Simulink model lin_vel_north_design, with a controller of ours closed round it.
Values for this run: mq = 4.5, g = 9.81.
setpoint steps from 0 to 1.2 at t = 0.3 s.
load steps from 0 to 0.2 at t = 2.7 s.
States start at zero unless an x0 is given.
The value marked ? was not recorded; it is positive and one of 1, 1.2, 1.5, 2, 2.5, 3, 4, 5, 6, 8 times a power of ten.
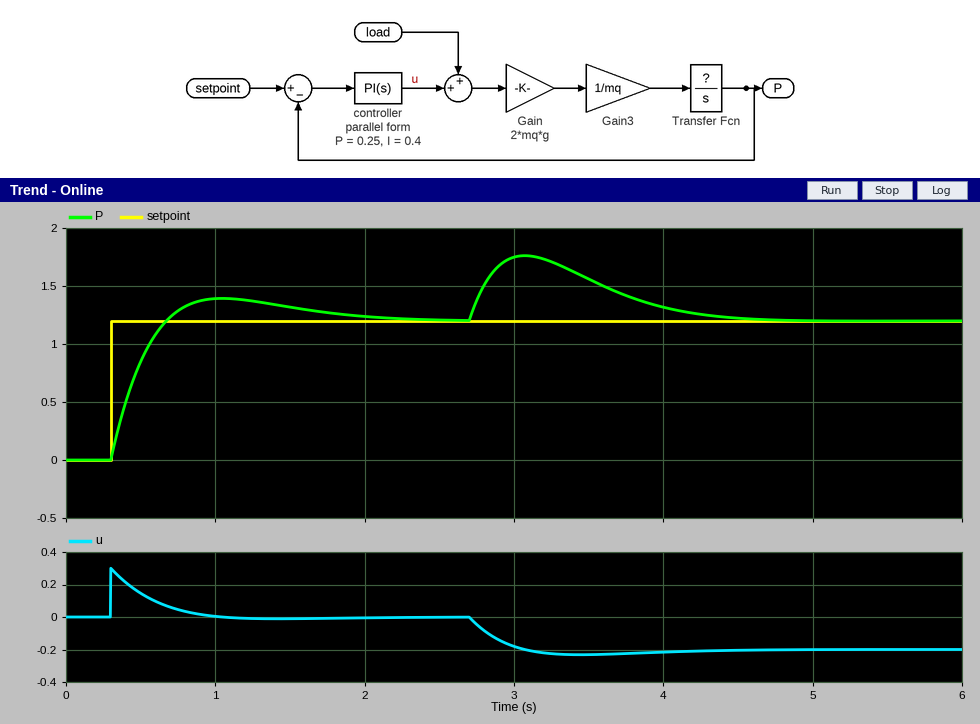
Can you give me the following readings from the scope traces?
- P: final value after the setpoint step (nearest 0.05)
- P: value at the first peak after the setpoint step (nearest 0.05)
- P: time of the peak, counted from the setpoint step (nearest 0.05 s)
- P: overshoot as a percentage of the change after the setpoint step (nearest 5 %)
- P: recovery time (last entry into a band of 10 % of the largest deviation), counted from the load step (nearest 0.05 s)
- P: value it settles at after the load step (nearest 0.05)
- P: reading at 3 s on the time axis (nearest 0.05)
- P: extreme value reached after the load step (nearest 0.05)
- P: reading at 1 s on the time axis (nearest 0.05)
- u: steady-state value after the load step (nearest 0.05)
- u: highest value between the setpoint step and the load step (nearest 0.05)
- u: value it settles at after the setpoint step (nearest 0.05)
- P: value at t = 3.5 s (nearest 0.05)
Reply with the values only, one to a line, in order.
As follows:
1.20
1.40
0.75 s
15 %
1.55 s
1.20
1.75
1.75
1.40
-0.20
0.30
0.00
1.55
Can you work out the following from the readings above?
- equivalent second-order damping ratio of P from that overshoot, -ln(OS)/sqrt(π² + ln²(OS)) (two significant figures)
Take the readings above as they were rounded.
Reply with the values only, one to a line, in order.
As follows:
0.52
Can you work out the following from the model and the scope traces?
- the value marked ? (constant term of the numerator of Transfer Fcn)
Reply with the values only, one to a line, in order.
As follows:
1
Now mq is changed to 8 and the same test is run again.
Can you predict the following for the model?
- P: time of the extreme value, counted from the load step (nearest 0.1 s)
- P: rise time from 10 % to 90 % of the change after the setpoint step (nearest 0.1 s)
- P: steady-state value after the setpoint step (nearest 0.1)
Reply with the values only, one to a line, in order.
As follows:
0.4 s
0.3 s
1.2
